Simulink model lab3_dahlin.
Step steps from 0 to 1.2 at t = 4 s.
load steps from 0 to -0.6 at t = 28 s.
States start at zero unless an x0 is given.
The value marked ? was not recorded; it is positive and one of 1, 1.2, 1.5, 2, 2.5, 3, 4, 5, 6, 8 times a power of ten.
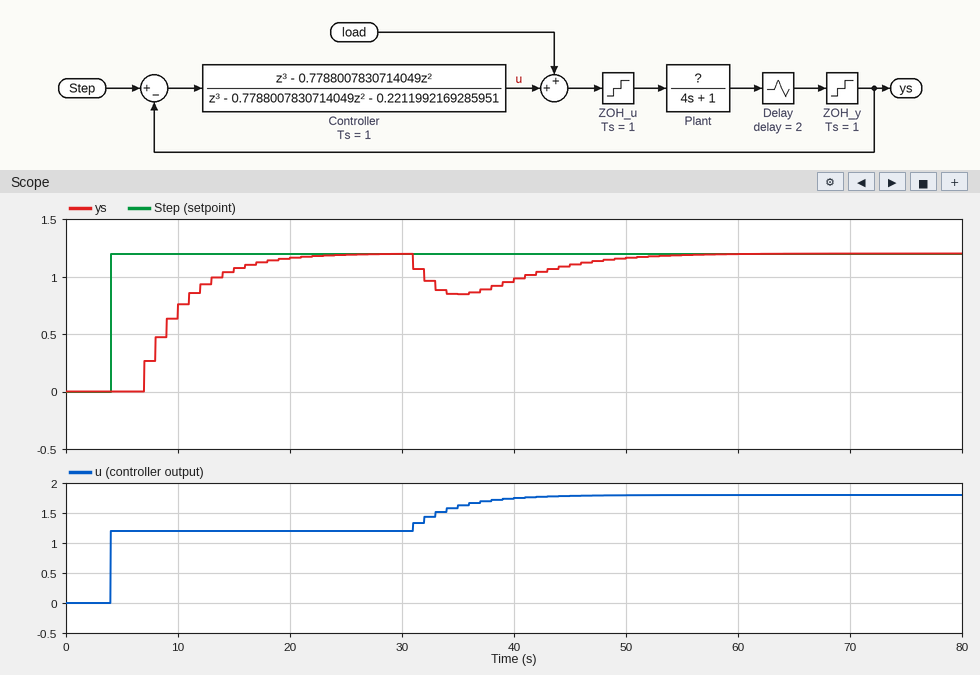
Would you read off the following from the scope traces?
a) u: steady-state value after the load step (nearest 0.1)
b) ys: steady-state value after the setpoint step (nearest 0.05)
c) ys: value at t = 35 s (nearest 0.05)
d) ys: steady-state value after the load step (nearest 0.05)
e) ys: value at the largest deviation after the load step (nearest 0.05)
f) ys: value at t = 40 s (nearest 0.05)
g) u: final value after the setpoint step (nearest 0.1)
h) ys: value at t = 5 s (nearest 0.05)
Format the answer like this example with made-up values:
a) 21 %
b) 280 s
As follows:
a) 1.8
b) 1.20
c) 0.85
d) 1.20
e) 0.85
f) 1.00
g) 1.2
h) 0.00
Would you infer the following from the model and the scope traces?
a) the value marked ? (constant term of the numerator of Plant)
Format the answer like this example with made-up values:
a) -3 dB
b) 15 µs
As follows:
a) 1
